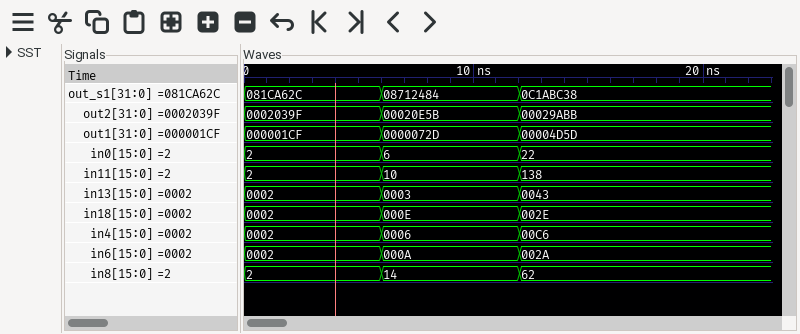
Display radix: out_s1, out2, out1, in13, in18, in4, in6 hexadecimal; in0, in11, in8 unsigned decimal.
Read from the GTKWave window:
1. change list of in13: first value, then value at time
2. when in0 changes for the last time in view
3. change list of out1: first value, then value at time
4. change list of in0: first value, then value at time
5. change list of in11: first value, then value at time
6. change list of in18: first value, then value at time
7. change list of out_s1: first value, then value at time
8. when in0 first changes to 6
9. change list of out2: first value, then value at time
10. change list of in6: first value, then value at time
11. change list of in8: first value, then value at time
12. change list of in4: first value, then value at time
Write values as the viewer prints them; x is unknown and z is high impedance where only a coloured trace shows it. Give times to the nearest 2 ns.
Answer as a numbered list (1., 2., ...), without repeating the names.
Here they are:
1. 0002, 0003 at 6 ns, 0043 at 12 ns
2. 12 ns
3. 000001CF, 0000072D at 6 ns, 00004D5D at 12 ns
4. 2, 6 at 6 ns, 22 at 12 ns
5. 2, 10 at 6 ns, 138 at 12 ns
6. 0002, 000E at 6 ns, 002E at 12 ns
7. 081CA62C, 08712484 at 6 ns, 0C1ABC38 at 12 ns
8. 6 ns
9. 0002039F, 00020E5B at 6 ns, 00029ABB at 12 ns
10. 0002, 000A at 6 ns, 002A at 12 ns
11. 2, 14 at 6 ns, 62 at 12 ns
12. 0002, 0006 at 6 ns, 00C6 at 12 ns
